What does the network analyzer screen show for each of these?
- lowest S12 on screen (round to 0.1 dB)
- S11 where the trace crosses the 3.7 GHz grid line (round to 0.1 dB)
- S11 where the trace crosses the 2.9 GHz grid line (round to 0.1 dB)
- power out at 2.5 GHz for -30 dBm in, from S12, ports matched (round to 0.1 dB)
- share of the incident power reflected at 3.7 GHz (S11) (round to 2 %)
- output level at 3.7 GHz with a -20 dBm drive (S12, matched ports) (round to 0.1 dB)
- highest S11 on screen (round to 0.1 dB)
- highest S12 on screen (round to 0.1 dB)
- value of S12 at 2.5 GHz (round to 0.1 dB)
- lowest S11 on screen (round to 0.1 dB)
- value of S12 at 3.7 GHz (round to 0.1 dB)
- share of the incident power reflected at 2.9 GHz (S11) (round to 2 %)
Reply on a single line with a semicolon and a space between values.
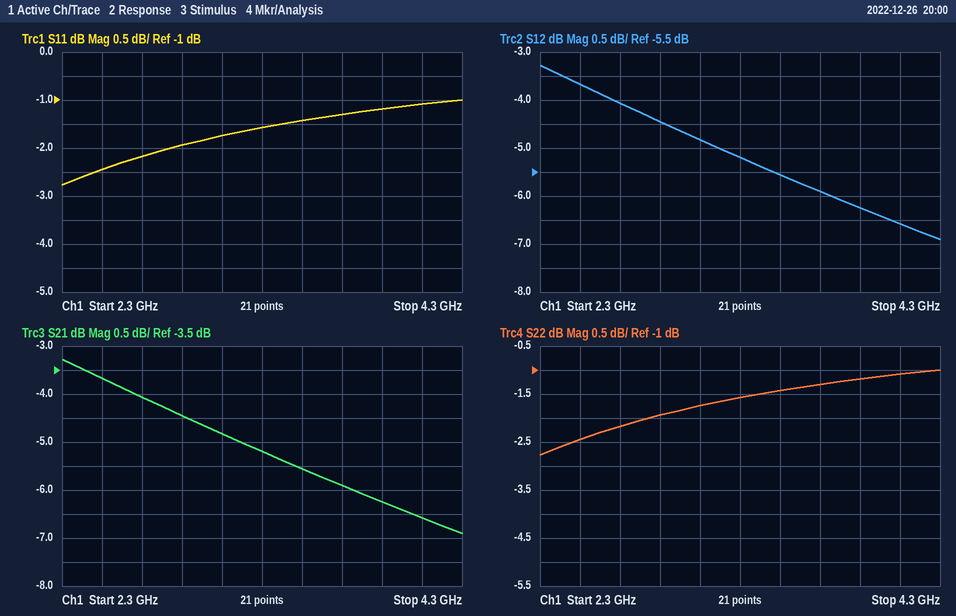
-6.9 dB; -1.3 dB; -1.9 dB; -33.7 dBm; 74 %; -25.9 dBm; -1.0 dB; -3.3 dB; -3.7 dB; -2.8 dB; -5.9 dB; 64 %
